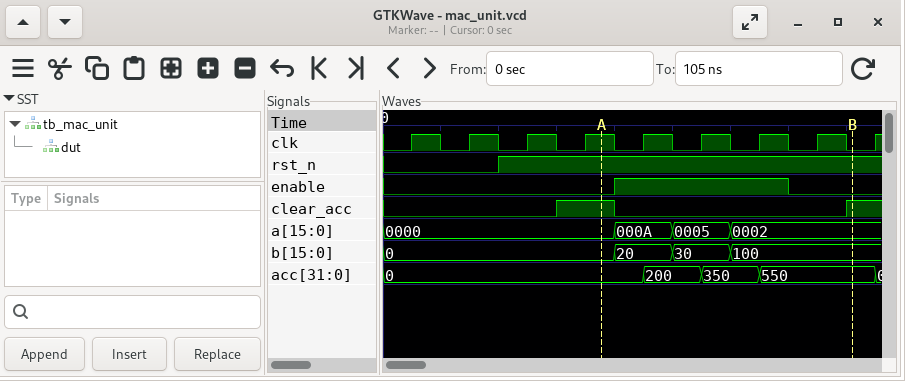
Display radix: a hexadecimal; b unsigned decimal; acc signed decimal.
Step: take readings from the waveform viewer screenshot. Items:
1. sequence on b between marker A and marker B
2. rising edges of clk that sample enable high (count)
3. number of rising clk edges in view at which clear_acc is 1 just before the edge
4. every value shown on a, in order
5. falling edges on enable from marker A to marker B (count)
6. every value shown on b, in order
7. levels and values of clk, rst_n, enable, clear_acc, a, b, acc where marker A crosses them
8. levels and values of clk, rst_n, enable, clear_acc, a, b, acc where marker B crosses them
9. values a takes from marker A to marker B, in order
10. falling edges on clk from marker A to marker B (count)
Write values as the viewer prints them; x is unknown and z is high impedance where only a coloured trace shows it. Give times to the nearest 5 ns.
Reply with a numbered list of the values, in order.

1. 0, 20, 30, 100
2. 3
3. 2
4. 0000, 000A, 0005, 0002
5. 1
6. 0, 20, 30, 100
7. clk=1, rst_n=1, enable=0, clear_acc=1, a=0000, b=0, acc=0
8. clk=0, rst_n=1, enable=0, clear_acc=1, a=0002, b=100, acc=550
9. 0000, 000A, 0005, 0002
10. 5
